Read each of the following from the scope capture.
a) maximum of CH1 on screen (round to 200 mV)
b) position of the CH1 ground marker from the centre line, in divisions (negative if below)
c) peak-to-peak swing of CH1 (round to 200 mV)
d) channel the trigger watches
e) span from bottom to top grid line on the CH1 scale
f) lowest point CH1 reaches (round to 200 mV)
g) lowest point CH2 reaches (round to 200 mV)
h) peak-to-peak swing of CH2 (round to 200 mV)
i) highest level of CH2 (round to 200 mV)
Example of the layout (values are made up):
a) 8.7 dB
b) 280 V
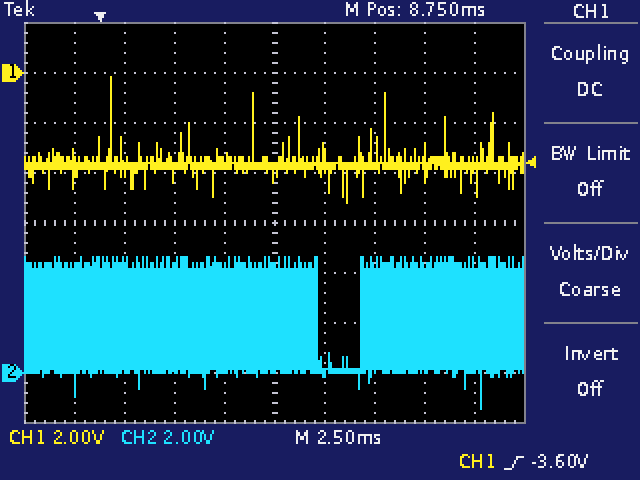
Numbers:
a) -200 mV
b) +3.0 div
c) 5.0 V
d) CH1
e) 16 V
f) -5.2 V
g) -1.4 V
h) 6.0 V
i) 4.6 V
